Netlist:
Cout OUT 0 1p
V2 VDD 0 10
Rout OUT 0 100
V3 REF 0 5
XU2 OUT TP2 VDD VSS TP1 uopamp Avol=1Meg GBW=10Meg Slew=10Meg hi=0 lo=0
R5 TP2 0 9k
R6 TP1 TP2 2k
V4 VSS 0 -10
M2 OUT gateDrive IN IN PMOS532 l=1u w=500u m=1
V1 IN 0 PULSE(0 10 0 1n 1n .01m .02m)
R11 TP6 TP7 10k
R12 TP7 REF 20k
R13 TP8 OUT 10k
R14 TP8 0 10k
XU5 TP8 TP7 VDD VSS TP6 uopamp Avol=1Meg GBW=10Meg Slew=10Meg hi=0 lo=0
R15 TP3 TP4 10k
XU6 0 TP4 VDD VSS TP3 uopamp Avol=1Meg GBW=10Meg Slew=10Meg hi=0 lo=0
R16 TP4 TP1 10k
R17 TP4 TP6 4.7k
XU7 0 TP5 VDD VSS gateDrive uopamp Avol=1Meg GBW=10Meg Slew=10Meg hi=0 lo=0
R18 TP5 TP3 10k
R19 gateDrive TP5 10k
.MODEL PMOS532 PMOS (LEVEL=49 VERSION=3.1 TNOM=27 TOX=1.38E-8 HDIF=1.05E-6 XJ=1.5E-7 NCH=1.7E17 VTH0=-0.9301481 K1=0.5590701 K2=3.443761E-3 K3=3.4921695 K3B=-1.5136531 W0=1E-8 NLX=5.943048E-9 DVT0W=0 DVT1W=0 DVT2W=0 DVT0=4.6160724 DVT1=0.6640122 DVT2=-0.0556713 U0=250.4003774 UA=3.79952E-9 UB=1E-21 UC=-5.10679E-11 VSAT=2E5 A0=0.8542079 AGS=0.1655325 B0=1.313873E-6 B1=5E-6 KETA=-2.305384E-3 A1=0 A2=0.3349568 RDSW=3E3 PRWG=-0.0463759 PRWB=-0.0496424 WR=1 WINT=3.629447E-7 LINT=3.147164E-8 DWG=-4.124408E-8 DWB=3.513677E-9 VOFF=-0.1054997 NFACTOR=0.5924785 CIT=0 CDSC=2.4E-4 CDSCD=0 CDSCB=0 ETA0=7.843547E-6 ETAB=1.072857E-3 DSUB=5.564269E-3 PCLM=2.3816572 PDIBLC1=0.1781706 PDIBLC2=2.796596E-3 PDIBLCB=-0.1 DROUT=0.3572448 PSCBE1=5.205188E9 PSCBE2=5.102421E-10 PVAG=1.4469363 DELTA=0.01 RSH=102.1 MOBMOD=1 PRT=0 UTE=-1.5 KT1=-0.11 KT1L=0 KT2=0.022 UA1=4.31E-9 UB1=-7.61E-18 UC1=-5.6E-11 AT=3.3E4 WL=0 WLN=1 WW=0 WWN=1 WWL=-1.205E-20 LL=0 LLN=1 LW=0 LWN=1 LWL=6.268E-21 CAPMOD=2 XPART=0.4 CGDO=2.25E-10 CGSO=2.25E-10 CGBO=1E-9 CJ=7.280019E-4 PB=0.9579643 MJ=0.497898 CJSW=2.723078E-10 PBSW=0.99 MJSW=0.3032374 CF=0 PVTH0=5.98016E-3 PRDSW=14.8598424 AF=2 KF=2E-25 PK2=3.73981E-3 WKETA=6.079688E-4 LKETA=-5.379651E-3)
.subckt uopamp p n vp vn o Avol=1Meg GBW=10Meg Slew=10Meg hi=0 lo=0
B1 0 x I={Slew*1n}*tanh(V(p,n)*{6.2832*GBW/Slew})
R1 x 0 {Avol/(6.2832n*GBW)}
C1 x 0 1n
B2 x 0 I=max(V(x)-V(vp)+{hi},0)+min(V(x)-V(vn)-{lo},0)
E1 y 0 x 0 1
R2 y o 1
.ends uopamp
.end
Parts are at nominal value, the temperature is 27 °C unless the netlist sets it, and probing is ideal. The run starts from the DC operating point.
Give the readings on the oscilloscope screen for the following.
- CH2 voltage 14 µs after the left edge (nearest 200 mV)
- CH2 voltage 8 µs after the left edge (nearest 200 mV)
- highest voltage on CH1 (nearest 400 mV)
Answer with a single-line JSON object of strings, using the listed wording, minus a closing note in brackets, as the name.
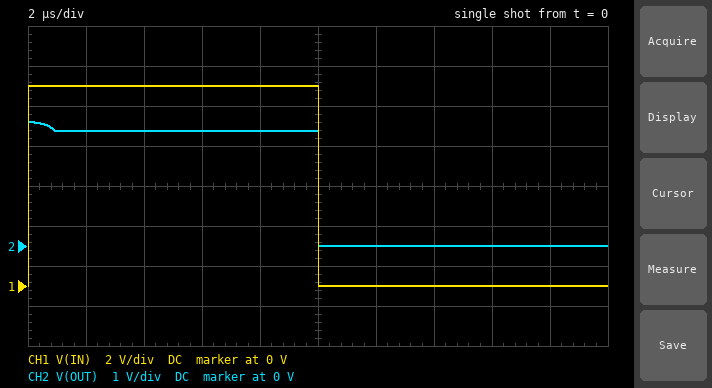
{"CH2 voltage 14 µs after the left edge": "0 V", "CH2 voltage 8 µs after the left edge": "2.8 V", "highest voltage on CH1": "10.0 V"}
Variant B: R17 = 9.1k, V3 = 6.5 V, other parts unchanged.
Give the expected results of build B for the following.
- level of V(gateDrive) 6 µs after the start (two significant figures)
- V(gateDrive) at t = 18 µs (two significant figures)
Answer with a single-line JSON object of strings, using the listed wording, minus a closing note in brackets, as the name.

{"level of V(gateDrive) 6 µs after the start": "2.4 V", "V(gateDrive) at t = 18 µs": "-3.6 V"}
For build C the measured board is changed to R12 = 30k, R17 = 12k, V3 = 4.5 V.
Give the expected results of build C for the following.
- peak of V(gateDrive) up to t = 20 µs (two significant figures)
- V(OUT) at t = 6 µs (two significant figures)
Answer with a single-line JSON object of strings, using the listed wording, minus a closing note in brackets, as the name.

{"peak of V(gateDrive) up to t = 20 µs": "3.6 V", "V(OUT) at t = 6 µs": "2.7 V"}
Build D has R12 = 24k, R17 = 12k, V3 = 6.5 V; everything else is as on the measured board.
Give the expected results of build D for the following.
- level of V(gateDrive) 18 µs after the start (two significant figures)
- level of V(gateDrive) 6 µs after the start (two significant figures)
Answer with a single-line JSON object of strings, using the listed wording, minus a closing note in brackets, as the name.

{"level of V(gateDrive) 18 µs after the start": "-2.3 V", "level of V(gateDrive) 6 µs after the start": "2.9 V"}
